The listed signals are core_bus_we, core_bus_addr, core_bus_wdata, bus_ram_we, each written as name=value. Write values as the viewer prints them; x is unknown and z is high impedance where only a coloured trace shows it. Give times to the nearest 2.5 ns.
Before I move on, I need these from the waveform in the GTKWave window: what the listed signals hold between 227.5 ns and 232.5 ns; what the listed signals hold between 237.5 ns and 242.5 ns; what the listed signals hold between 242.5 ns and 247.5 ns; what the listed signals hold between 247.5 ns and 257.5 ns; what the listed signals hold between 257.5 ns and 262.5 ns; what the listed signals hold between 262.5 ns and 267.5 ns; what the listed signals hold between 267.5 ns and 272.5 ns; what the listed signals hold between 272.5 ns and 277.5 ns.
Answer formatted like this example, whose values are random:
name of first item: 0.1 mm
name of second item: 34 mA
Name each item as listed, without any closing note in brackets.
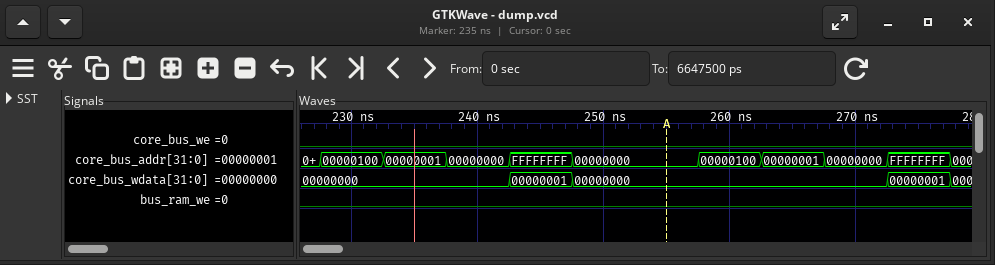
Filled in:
what the listed signals hold between 227.5 ns and 232.5 ns: core_bus_we=0, core_bus_addr=00000100, core_bus_wdata=00000000, bus_ram_we=0
what the listed signals hold between 237.5 ns and 242.5 ns: core_bus_we=0, core_bus_addr=00000000, core_bus_wdata=00000000, bus_ram_we=0
what the listed signals hold between 242.5 ns and 247.5 ns: core_bus_we=0, core_bus_addr=FFFFFFFF, core_bus_wdata=00000001, bus_ram_we=0
what the listed signals hold between 247.5 ns and 257.5 ns: core_bus_we=0, core_bus_addr=00000000, core_bus_wdata=00000000, bus_ram_we=0
what the listed signals hold between 257.5 ns and 262.5 ns: core_bus_we=0, core_bus_addr=00000100, core_bus_wdata=00000000, bus_ram_we=0
what the listed signals hold between 262.5 ns and 267.5 ns: core_bus_we=0, core_bus_addr=00000001, core_bus_wdata=00000000, bus_ram_we=0
what the listed signals hold between 267.5 ns and 272.5 ns: core_bus_we=0, core_bus_addr=00000000, core_bus_wdata=00000000, bus_ram_we=0
what the listed signals hold between 272.5 ns and 277.5 ns: core_bus_we=0, core_bus_addr=FFFFFFFF, core_bus_wdata=00000001, bus_ram_we=0
